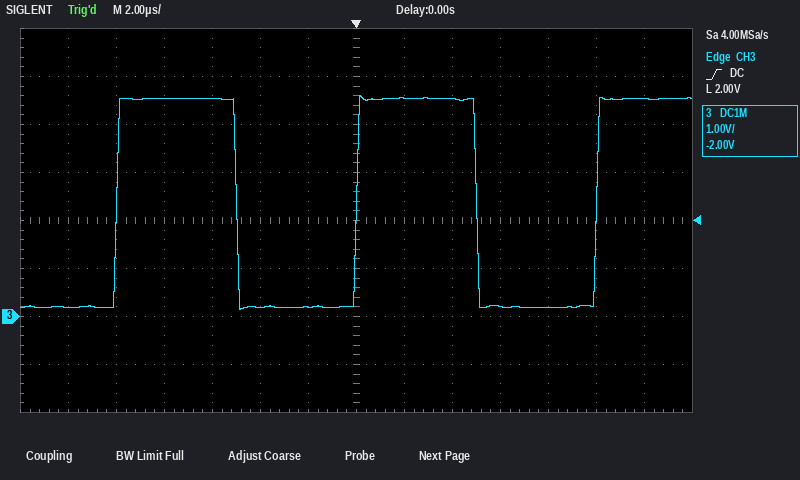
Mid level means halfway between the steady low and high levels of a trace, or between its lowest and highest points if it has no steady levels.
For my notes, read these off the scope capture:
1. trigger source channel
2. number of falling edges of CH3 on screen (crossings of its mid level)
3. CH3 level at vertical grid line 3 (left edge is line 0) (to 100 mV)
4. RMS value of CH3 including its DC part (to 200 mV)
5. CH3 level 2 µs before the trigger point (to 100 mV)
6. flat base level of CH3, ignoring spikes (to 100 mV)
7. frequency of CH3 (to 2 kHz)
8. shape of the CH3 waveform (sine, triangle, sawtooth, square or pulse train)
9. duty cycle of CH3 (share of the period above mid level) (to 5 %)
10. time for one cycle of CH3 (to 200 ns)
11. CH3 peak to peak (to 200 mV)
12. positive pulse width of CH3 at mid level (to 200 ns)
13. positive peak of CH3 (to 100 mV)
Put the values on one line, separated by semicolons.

CH3; 2; 4.5 V; 3.2 V; 200 mV; 200 mV; 100 kHz; square; 50 %; 10.0 µs; 4.4 V; 5.0 µs; 4.6 V
